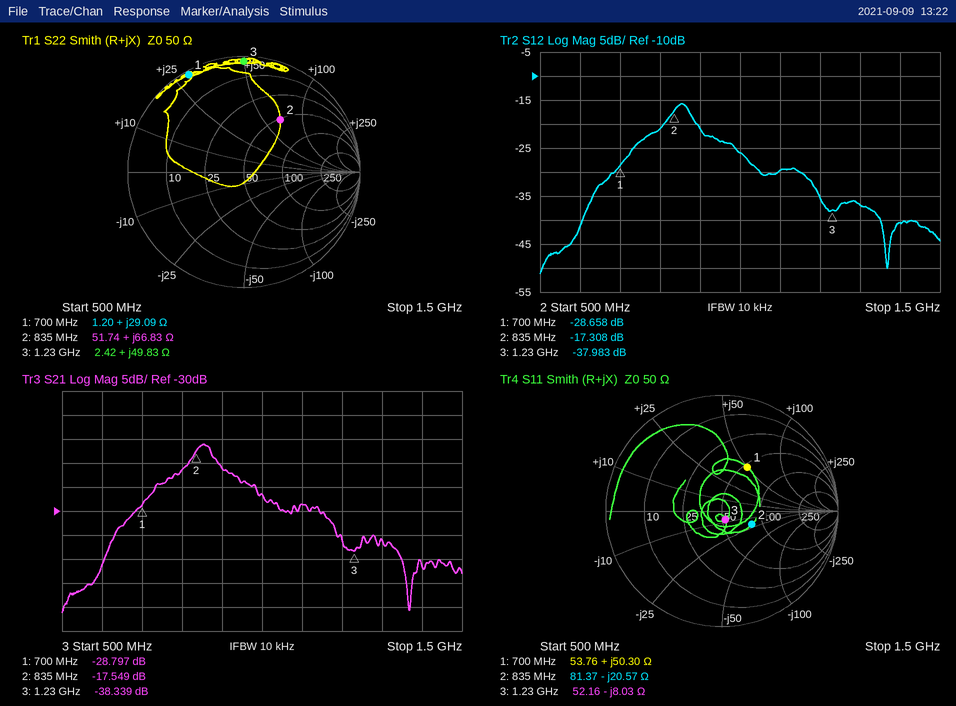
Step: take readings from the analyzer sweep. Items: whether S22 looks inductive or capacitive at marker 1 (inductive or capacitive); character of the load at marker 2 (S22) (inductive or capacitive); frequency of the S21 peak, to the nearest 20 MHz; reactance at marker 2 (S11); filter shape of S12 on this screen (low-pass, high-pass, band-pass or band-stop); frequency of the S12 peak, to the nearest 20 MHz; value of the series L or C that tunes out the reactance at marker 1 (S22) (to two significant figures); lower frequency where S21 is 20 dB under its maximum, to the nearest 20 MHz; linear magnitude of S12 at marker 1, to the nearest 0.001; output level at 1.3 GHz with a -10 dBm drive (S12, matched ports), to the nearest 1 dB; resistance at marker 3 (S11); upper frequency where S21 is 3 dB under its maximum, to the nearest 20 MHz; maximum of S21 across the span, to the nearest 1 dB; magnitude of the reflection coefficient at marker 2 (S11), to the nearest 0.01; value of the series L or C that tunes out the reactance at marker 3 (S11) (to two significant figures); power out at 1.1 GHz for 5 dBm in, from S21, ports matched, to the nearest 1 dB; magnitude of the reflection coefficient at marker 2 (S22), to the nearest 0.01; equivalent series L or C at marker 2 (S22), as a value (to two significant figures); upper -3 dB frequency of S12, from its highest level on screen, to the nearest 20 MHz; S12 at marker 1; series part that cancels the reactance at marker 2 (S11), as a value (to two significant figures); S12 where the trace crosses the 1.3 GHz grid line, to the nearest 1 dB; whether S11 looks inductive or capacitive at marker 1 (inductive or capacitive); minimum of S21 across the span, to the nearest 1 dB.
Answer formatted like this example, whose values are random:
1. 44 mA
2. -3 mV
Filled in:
1. inductive
2. inductive
3. 860 MHz
4. -20.57 Ω
5. band-pass
6. 860 MHz
7. 7.8 pF
8. 620 MHz
9. 0.037
10. -47 dBm
11. 52.16 Ω
12. 880 MHz
13. -16 dB
14. 0.28
15. 1.0 nH
16. -24 dBm
17. 0.55
18. 13 nH
19. 880 MHz
20. -28.658 dB
21. 3.9 nH
22. -37 dB
23. inductive
24. -51 dB
